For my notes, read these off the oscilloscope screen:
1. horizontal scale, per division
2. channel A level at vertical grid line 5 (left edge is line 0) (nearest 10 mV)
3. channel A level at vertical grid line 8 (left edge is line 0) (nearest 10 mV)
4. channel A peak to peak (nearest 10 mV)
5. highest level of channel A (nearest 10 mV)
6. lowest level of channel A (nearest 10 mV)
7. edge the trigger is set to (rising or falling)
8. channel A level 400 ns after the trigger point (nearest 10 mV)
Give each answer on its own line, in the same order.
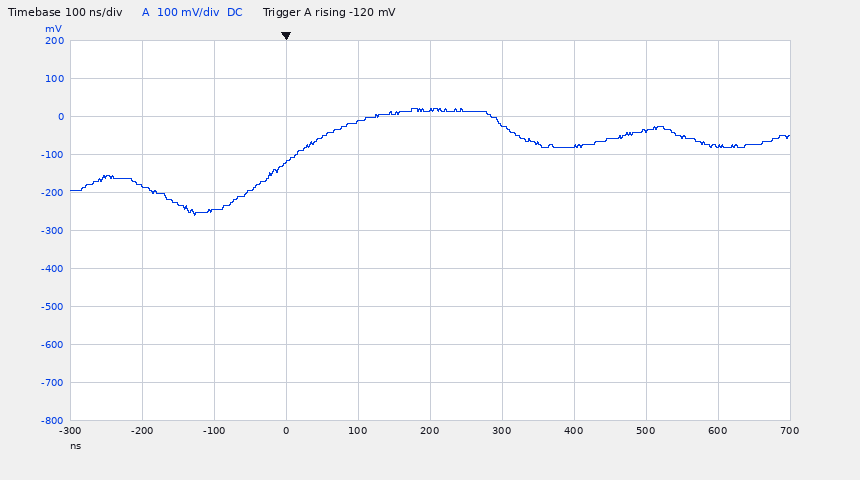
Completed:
100 ns
20 mV
-40 mV
280 mV
20 mV
-260 mV
rising
-80 mV
